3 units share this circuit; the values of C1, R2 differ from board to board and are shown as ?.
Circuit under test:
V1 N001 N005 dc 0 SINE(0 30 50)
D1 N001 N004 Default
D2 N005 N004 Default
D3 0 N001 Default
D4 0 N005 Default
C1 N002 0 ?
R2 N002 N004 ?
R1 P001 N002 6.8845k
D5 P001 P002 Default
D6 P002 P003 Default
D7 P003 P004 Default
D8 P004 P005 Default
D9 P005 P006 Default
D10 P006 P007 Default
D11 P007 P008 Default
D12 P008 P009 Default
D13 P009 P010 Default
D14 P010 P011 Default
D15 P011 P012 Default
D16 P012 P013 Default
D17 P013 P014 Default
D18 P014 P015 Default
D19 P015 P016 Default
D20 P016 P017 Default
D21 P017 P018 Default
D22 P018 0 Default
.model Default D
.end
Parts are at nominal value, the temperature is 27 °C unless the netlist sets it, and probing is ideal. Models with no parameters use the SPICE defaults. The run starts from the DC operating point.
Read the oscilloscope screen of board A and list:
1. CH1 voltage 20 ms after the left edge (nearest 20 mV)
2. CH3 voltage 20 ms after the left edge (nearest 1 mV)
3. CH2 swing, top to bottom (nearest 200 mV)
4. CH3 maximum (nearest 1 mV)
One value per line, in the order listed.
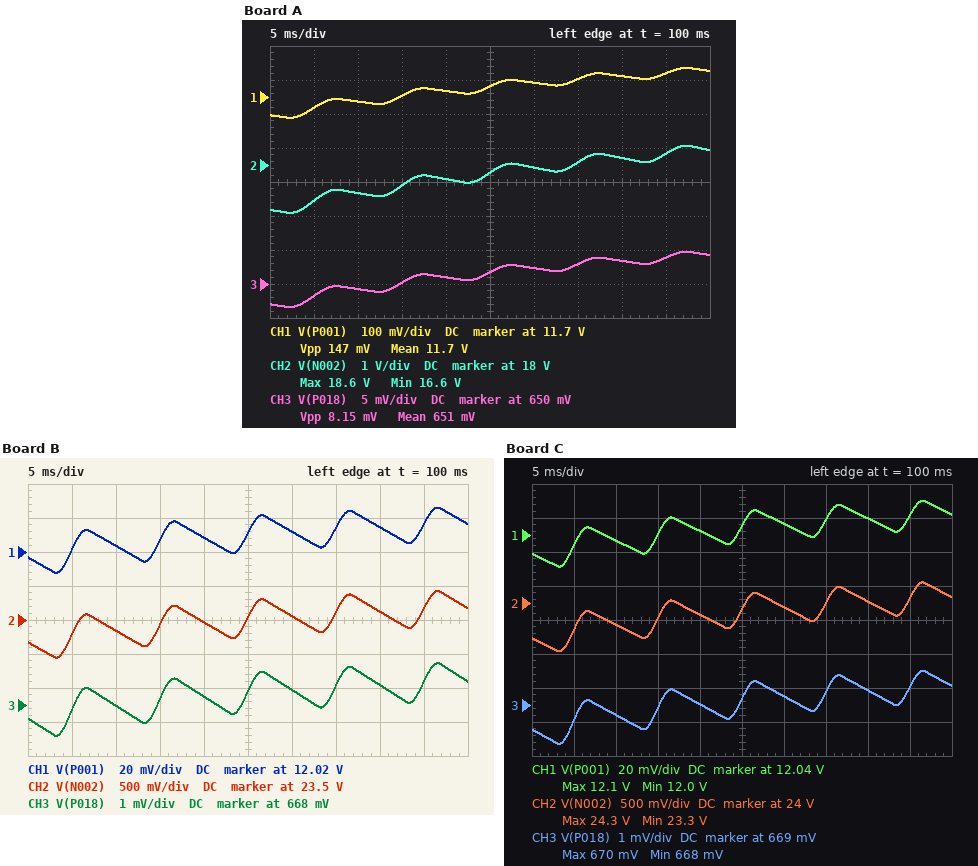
11.72 V
651 mV
2.0 V
655 mV
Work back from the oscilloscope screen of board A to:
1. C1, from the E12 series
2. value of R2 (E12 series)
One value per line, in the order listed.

18 µF
2.7 kΩ
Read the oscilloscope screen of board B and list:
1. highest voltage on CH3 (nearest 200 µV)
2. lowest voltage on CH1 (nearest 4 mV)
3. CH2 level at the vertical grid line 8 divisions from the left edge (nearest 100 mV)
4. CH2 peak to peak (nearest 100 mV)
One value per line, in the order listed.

669.2 mV
12.008 V
23.6 V
1.0 V
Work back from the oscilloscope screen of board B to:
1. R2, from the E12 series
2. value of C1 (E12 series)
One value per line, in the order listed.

680 Ω
22 µF
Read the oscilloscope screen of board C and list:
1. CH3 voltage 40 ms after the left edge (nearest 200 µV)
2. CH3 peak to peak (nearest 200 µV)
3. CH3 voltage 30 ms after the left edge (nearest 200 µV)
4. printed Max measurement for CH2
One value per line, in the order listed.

669.4 mV
2.2 mV
669.2 mV
24.3 V
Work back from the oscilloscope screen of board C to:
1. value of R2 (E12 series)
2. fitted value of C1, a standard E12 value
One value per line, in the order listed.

560 Ω
27 µF
